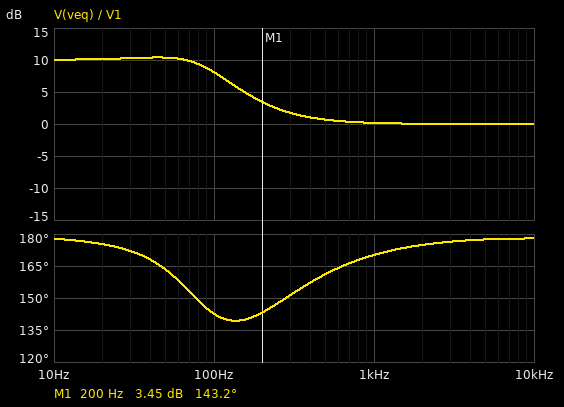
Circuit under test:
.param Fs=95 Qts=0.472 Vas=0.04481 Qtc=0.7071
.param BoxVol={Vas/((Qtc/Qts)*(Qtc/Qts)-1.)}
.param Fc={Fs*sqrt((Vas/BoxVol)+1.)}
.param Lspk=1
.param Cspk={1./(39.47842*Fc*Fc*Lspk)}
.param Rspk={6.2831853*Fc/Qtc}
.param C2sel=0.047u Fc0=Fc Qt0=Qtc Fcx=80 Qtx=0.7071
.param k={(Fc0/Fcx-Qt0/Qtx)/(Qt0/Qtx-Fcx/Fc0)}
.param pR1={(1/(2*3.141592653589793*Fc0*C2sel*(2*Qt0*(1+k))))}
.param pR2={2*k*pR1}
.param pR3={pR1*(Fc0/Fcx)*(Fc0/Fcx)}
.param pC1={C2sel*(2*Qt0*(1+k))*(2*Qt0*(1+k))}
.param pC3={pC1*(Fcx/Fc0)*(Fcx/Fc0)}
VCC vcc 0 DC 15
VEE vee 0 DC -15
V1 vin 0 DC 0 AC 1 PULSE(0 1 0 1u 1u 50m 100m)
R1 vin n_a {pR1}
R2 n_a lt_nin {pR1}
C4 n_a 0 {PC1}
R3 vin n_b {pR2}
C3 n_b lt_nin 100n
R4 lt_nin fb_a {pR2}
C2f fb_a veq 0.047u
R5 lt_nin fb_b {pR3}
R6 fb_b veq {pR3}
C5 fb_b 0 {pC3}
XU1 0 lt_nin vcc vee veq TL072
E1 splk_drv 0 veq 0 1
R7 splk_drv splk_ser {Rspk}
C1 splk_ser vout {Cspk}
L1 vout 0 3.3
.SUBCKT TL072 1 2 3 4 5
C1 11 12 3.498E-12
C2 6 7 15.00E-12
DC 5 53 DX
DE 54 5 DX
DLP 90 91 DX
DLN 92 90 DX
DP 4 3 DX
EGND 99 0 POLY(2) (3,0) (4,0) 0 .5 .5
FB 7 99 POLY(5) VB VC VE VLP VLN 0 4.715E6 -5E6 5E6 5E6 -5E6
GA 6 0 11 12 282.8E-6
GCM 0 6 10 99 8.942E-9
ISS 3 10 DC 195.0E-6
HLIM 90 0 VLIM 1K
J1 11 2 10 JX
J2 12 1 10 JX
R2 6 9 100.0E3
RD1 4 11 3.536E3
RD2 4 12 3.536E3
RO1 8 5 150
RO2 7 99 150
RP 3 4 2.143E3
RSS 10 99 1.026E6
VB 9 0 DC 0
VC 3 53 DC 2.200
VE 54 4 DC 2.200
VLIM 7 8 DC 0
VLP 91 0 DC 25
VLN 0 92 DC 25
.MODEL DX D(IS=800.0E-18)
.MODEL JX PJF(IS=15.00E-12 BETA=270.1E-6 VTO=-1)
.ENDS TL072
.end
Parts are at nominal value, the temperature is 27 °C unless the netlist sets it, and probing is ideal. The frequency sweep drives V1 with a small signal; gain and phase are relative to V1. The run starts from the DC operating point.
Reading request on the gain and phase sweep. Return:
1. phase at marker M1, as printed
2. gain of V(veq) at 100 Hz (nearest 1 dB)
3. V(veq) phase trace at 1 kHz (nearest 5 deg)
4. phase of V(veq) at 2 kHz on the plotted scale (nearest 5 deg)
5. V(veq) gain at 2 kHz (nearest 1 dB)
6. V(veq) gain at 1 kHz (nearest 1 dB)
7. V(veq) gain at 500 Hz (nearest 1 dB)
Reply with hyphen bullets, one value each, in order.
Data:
- 143.2 deg
- 8 dB
- 170 deg
- 175 deg
- 0 dB
- 0 dB
- 1 dB
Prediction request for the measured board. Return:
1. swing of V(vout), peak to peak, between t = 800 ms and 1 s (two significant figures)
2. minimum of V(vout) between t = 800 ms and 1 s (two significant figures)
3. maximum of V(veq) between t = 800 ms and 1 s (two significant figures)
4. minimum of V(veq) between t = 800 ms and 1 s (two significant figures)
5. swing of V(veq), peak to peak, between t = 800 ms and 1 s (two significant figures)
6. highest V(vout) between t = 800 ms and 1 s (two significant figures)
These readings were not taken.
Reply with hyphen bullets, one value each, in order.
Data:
- 2.7 V
- -1.3 V
- 220 mV
- -3.4 V
- 3.6 V
- 1.3 V
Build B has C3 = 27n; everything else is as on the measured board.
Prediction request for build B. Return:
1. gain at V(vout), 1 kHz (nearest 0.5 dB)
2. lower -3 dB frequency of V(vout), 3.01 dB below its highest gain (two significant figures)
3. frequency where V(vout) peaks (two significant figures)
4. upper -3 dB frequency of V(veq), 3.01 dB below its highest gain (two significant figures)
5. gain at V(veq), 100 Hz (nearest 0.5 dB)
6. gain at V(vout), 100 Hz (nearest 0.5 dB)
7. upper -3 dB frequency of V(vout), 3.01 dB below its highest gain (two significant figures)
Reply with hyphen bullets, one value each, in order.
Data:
- -0.5 dB
- 58 Hz
- 79 Hz
- 81 Hz
- 5.0 dB
- 7.5 dB
- 110 Hz
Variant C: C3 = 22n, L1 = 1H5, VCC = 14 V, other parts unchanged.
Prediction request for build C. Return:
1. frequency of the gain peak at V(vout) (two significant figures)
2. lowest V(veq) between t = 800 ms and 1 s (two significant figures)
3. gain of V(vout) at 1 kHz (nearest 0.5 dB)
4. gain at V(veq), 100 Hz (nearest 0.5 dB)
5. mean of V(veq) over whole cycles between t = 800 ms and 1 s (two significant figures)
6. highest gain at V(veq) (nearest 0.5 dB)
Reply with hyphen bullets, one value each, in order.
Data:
- 100 Hz
- -3.3 V
- -0.5 dB
- 5.0 dB
- -1.6 V
- 10.0 dB
